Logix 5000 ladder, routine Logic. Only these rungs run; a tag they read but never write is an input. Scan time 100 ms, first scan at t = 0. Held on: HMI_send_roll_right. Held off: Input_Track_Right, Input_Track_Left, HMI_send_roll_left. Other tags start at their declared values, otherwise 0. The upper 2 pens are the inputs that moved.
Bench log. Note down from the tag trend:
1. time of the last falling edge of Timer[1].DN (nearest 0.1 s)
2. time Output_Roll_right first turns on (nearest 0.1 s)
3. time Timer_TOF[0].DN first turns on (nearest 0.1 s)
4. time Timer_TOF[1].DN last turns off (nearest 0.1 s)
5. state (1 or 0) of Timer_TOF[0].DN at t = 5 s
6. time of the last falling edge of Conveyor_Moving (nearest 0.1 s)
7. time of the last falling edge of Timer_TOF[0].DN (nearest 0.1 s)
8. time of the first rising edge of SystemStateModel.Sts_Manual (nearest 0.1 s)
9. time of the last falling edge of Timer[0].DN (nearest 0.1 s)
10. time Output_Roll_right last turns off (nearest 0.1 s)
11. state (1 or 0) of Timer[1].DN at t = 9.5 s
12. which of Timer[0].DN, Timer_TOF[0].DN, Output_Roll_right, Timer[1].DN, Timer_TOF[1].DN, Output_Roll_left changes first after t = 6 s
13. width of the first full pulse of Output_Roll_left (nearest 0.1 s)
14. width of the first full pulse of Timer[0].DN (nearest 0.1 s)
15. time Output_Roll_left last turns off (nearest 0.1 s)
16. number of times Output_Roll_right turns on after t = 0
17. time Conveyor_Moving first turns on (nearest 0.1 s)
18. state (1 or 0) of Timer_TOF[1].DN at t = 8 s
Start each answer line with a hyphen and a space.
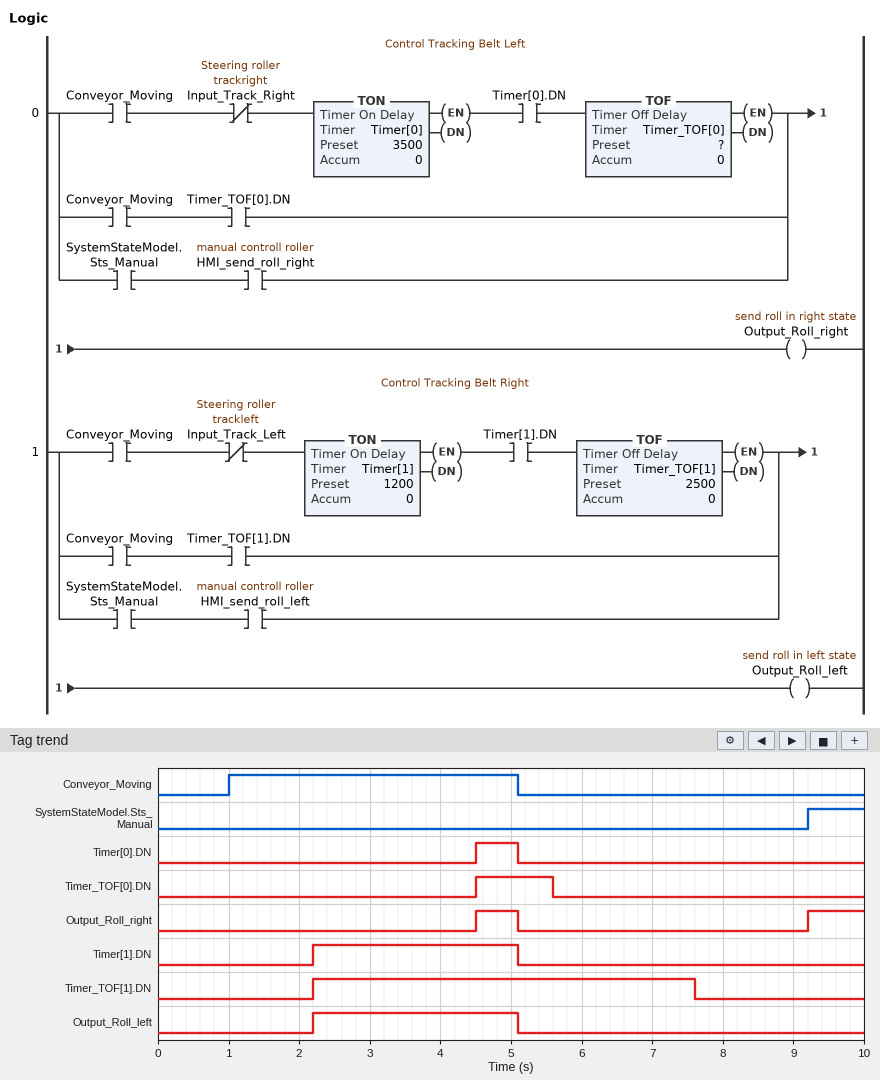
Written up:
- 5.1 s
- 4.5 s
- 4.5 s
- 7.6 s
- 1
- 5.1 s
- 5.6 s
- 9.2 s
- 5.1 s
- 5.1 s
- 0
- Timer_TOF[1].DN
- 2.9 s
- 0.6 s
- 5.1 s
- 2
- 1.0 s
- 0
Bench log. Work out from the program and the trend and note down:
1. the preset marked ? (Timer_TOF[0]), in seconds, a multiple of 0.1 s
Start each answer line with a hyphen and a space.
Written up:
- 0.5 s
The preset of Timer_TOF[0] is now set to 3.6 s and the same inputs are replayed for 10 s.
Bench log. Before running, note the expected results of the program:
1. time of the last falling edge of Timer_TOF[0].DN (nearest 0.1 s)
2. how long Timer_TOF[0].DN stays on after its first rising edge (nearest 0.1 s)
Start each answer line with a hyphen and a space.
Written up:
- 8.7 s
- 4.2 s
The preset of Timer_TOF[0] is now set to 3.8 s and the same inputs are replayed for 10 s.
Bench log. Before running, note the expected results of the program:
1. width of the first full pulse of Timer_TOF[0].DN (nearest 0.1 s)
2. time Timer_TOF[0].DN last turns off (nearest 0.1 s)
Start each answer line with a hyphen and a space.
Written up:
- 4.4 s
- 8.9 s
